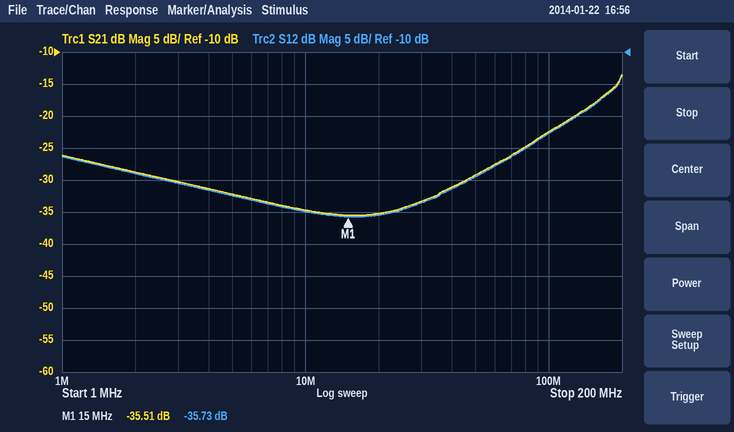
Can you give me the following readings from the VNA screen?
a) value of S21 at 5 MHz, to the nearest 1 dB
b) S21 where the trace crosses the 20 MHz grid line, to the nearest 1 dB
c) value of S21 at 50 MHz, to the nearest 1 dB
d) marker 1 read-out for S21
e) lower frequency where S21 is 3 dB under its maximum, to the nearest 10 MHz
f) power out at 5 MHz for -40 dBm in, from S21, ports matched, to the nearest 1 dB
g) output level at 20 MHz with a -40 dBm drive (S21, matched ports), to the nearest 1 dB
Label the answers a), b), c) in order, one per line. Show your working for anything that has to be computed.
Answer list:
a) -32 dB
b) -35 dB
c) -29 dB
d) -35.51 dB
e) 170 MHz
f) -40 dBm + (-32 dB) = -72 dBm
g) -40 dBm + (-35 dB) = -75 dBm
